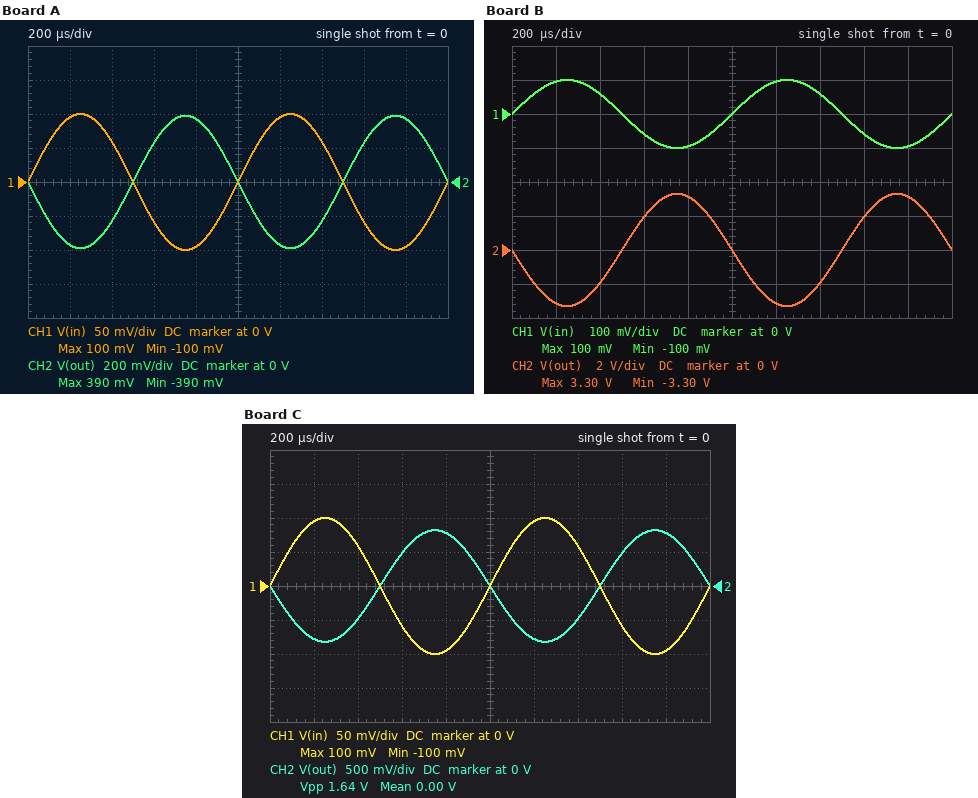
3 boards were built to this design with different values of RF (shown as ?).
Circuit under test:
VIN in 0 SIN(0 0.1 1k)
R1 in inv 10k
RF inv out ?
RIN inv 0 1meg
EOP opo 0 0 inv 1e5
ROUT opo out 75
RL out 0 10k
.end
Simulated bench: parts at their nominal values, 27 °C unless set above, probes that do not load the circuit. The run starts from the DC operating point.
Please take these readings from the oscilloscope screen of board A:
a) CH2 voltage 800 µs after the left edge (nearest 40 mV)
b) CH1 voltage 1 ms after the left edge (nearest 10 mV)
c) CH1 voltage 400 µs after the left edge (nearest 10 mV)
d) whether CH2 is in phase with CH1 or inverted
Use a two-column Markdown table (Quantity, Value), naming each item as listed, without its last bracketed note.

| Quantity | Value |
|---|---|
| CH2 voltage 800 µs after the left edge | 360 mV |
| CH1 voltage 1 ms after the left edge | 0 V |
| CH1 voltage 400 µs after the left edge | 60 mV |
| whether CH2 is in phase with CH1 or inverted | inverted |
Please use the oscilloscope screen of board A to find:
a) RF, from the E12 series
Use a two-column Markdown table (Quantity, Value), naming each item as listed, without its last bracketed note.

| Quantity | Value |
|---|---|
| RF, from the E12 series | 39 kΩ |
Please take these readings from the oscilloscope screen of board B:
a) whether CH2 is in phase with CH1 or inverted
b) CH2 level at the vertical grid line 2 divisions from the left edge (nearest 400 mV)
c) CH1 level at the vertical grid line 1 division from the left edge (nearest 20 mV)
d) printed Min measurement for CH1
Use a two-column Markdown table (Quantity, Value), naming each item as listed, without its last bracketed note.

| Quantity | Value |
|---|---|
| whether CH2 is in phase with CH1 or inverted | inverted |
| CH2 level at the vertical grid line 2 divisions from the left edge | -2.0 V |
| CH1 level at the vertical grid line 1 division from the left edge | 100 mV |
| printed Min measurement for CH1 | -100 mV |
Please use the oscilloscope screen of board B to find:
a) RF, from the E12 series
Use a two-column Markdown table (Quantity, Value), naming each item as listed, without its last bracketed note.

| Quantity | Value |
|---|---|
| RF, from the E12 series | 330 kΩ |
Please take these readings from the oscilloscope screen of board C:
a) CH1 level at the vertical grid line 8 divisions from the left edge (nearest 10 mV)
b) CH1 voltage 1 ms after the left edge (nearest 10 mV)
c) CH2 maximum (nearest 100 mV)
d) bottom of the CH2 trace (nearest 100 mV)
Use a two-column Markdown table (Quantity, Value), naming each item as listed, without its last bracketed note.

| Quantity | Value |
|---|---|
| CH1 level at the vertical grid line 8 divisions from the left edge | -60 mV |
| CH1 voltage 1 ms after the left edge | 0 V |
| CH2 maximum | 800 mV |
| bottom of the CH2 trace | -800 mV |
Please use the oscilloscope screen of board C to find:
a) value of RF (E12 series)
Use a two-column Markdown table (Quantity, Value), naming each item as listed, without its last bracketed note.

| Quantity | Value |
|---|---|
| value of RF | 82 kΩ |
